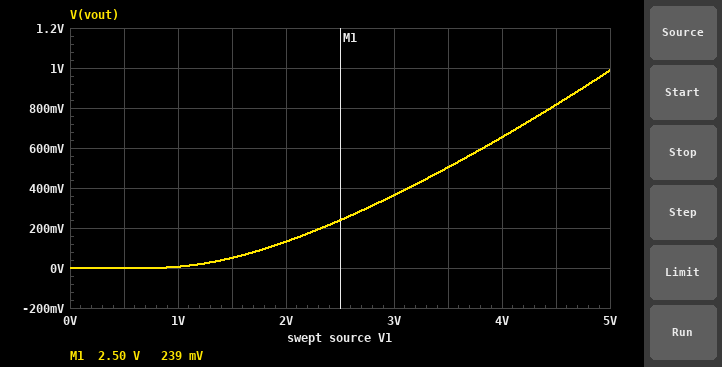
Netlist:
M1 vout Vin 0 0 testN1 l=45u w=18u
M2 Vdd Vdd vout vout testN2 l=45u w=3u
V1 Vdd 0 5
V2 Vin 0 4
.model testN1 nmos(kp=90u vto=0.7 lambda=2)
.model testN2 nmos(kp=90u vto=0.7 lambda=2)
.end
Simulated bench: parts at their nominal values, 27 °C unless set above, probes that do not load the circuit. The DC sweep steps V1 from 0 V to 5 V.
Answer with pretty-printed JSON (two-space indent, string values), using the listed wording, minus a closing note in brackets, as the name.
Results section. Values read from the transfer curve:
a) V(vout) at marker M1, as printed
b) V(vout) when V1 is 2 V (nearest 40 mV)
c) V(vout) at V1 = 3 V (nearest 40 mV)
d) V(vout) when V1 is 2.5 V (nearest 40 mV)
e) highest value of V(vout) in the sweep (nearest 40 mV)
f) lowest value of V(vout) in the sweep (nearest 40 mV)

{
  "V(vout) at marker M1, as printed": "239 mV",
  "V(vout) when V1 is 2 V": "120 mV",
  "V(vout) at V1 = 3 V": "360 mV",
  "V(vout) when V1 is 2.5 V": "240 mV",
  "highest value of V(vout) in the sweep": "1.00 V",
  "lowest value of V(vout) in the sweep": "0 V"
}
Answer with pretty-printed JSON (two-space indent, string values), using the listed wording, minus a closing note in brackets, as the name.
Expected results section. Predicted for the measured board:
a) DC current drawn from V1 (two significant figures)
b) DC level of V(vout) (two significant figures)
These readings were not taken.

{
  "DC current drawn from V1": "300 µA",
  "DC level of V(vout)": "990 mV"
}
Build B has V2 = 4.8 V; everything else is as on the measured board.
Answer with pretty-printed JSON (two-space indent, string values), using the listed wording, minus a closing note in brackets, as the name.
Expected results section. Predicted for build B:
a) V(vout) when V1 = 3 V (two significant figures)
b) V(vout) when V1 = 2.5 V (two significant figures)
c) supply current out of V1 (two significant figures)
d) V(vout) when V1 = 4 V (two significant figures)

{
  "V(vout) when V1 = 3 V": "320 mV",
  "V(vout) when V1 = 2.5 V": "210 mV",
  "supply current out of V1": "320 µA",
  "V(vout) when V1 = 4 V": "580 mV"
}
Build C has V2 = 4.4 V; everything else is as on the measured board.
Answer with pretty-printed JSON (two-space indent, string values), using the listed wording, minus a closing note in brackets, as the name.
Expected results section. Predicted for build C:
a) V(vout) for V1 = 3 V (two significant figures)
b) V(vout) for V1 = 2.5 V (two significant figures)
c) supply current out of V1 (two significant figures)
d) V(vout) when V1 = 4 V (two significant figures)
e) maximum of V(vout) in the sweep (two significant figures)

{
  "V(vout) for V1 = 3 V": "340 mV",
  "V(vout) for V1 = 2.5 V": "220 mV",
  "supply current out of V1": "310 µA",
  "V(vout) when V1 = 4 V": "620 mV",
  "maximum of V(vout) in the sweep": "930 mV"
}
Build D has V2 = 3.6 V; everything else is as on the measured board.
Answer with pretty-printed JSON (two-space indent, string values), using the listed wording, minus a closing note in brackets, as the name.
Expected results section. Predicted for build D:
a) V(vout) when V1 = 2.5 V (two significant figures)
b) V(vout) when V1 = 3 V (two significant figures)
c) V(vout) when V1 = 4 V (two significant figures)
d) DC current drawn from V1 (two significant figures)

{
  "V(vout) when V1 = 2.5 V": "260 mV",
  "V(vout) when V1 = 3 V": "390 mV",
  "V(vout) when V1 = 4 V": "700 mV",
  "DC current drawn from V1": "280 µA"
}
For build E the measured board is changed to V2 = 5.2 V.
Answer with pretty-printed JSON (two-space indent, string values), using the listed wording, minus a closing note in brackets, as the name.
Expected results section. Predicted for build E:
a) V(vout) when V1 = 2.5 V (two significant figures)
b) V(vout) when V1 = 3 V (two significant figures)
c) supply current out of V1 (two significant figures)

{
  "V(vout) when V1 = 2.5 V": "200 mV",
  "V(vout) when V1 = 3 V": "300 mV",
  "supply current out of V1": "330 µA"
}
